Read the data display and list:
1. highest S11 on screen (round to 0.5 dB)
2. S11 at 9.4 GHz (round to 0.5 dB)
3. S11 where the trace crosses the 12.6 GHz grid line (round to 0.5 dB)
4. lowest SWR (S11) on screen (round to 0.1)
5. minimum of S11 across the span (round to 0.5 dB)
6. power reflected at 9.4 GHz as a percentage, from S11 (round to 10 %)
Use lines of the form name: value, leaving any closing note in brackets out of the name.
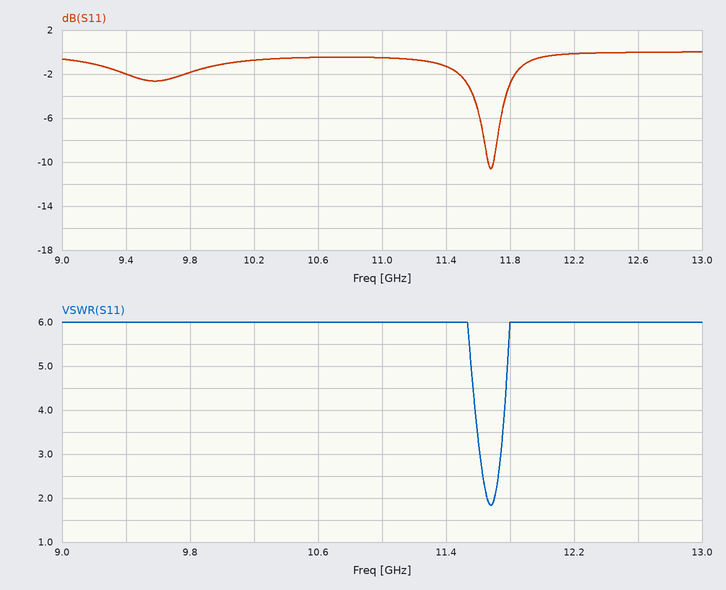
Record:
highest S11 on screen: 0.0 dB
S11 at 9.4 GHz: -2.0 dB
S11 where the trace crosses the 12.6 GHz grid line: 0.0 dB
lowest SWR (S11) on screen: 1.8
minimum of S11 across the span: -10.5 dB
power reflected at 9.4 GHz as a percentage, from S11: 60 %
